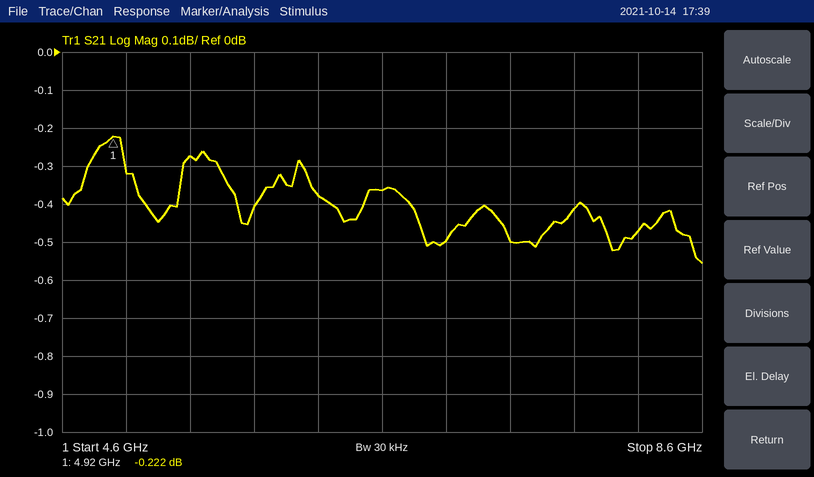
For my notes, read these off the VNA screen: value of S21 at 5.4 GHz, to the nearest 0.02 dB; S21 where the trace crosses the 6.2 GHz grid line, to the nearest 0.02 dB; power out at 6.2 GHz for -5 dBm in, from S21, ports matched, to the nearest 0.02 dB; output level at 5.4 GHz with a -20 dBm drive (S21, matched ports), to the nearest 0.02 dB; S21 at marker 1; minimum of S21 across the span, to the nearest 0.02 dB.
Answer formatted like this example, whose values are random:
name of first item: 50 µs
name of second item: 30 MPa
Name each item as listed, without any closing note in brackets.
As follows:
value of S21 at 5.4 GHz, to the nearest 0.02 dB: -0.28 dB
S21 where the trace crosses the 6.2 GHz grid line, to the nearest 0.02 dB: -0.38 dB
power out at 6.2 GHz for -5 dBm in, from S21, ports matched, to the nearest 0.02 dB: -5.38 dBm
output level at 5.4 GHz with a -20 dBm drive (S21, matched ports), to the nearest 0.02 dB: -20.28 dBm
S21 at marker 1: -0.222 dB
minimum of S21 across the span, to the nearest 0.02 dB: -0.56 dB
